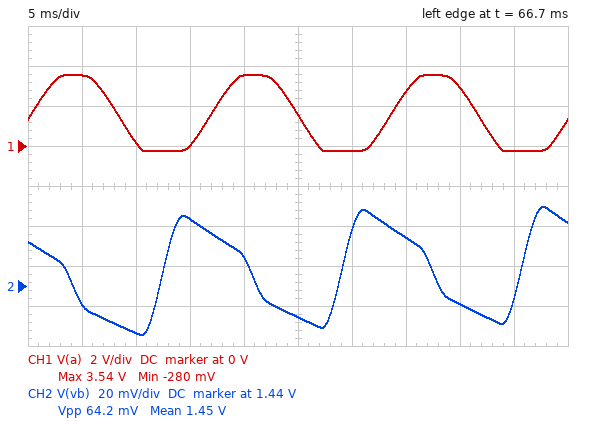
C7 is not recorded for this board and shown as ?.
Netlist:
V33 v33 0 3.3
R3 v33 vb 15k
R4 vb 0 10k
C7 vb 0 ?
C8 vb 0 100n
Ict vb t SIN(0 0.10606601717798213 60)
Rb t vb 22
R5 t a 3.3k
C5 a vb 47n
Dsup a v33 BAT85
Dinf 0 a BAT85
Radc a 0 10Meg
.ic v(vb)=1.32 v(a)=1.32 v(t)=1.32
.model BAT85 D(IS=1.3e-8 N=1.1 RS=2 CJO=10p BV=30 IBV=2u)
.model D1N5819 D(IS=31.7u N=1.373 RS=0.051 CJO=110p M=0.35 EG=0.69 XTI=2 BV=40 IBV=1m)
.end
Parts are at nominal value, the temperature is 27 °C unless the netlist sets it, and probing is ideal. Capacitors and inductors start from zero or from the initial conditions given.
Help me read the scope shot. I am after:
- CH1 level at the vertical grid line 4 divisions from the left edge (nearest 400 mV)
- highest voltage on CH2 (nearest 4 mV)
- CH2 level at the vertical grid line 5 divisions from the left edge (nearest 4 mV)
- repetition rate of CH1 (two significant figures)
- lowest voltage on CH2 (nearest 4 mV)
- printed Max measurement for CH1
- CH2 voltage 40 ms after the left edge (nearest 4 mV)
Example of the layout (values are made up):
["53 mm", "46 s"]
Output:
["3.6 V", "1.480 V", "1.424 V", "60 Hz", "1.416 V", "3.54 V", "1.432 V"]
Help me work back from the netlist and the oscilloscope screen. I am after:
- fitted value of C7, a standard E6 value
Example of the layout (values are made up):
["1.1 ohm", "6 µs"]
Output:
["6.8 µF"]
